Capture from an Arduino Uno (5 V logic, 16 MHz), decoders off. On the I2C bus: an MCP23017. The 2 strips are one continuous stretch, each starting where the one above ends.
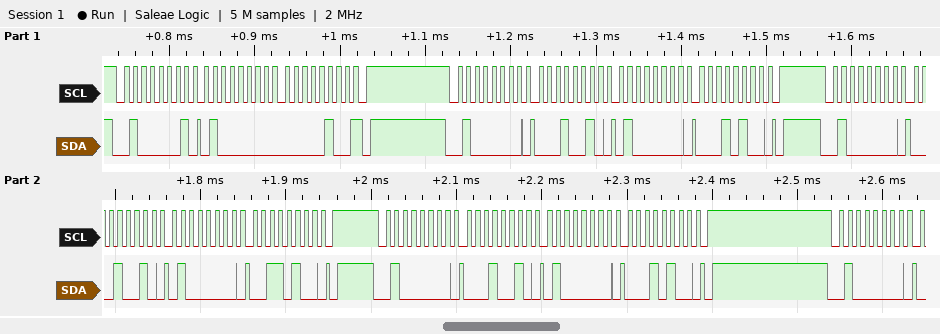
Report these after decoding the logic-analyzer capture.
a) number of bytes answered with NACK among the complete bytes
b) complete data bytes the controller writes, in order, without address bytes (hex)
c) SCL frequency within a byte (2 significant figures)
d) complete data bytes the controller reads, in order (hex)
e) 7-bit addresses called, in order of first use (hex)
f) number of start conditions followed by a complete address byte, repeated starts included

1
12 40 14 12 40 34 12 40 14
100 kHz
40 04
0x20
5
